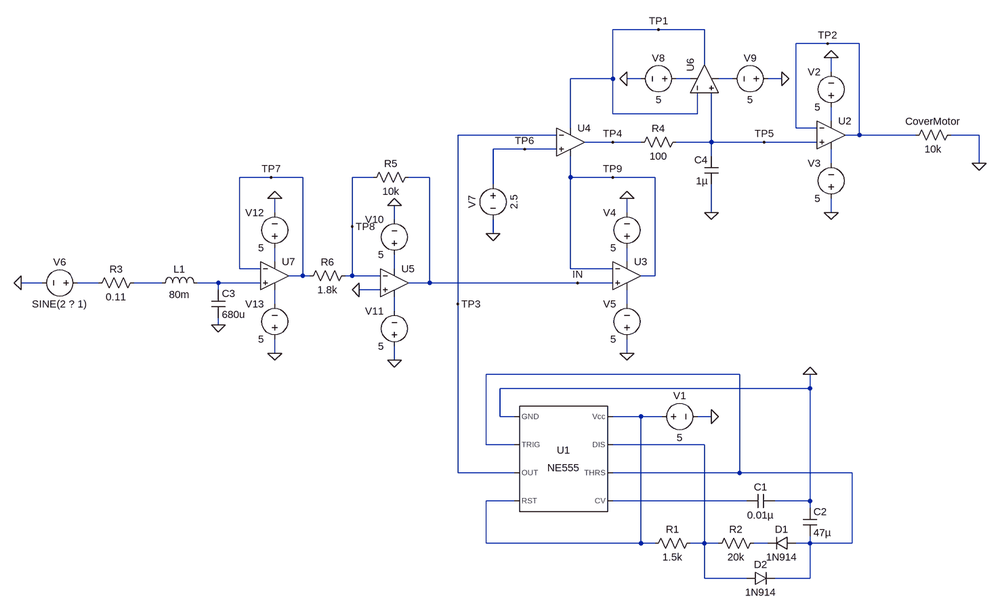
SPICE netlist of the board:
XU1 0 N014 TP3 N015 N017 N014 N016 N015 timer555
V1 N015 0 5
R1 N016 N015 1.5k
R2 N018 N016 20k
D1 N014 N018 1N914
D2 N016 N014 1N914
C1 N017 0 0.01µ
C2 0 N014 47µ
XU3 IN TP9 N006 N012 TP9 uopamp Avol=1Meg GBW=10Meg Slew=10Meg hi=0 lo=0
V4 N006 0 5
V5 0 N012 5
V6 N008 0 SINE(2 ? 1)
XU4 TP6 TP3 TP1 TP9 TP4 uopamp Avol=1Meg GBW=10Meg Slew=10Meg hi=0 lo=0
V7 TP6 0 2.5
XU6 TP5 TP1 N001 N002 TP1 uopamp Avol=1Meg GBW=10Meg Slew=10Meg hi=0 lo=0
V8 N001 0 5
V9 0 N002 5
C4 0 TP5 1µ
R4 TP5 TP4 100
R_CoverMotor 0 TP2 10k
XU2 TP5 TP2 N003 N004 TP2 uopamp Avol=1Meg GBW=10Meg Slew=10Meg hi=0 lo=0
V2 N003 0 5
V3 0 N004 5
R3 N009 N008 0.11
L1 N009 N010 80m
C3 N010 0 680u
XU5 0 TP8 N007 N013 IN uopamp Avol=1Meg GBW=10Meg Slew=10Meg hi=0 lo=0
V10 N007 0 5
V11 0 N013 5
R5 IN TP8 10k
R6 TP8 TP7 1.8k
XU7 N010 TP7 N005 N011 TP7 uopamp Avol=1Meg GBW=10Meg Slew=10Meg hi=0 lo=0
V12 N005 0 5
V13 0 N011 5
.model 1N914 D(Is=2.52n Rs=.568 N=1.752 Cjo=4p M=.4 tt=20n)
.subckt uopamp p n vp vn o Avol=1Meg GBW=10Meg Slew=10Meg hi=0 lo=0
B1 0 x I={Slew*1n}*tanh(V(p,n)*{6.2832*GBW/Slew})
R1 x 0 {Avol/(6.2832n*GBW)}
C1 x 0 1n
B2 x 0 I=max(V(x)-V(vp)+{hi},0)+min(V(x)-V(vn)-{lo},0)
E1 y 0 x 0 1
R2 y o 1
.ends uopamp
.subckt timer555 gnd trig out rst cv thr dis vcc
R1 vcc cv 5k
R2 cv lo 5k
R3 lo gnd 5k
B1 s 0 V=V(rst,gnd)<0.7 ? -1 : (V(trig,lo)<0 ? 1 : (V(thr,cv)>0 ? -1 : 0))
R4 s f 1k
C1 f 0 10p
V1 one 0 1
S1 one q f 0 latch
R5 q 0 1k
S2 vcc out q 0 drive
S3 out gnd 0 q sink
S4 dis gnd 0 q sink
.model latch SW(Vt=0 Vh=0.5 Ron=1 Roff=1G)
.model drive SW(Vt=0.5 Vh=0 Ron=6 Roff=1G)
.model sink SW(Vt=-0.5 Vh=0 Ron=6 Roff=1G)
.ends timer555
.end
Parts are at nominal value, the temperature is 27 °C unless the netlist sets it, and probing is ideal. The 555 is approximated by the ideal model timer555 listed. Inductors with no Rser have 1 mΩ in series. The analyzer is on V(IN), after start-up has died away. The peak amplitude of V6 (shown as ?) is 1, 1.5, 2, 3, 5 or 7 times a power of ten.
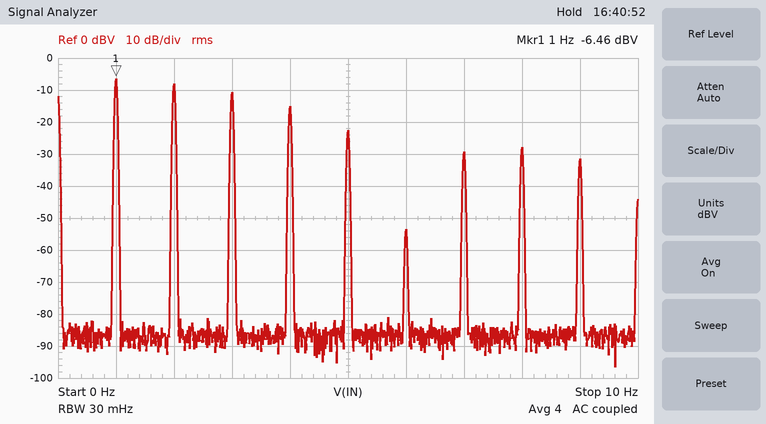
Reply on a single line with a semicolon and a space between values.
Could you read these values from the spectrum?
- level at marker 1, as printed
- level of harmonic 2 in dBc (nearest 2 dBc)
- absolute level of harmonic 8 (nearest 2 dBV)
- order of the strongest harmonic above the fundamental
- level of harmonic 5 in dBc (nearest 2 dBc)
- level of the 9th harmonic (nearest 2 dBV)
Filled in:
-6.46 dBV; -2 dBc; -28 dBV; 2; -16 dBc; -32 dBV
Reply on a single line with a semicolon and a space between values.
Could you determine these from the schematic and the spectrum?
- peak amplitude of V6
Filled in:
1.5 V
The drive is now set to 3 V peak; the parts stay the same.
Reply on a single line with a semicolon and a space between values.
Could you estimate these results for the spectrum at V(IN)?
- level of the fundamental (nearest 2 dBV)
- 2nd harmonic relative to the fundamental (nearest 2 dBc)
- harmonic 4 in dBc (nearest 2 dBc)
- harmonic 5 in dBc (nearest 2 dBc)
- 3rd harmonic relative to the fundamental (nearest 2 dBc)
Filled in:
10 dBV; -4 dBc; -28 dBc; -20 dBc; -14 dBc
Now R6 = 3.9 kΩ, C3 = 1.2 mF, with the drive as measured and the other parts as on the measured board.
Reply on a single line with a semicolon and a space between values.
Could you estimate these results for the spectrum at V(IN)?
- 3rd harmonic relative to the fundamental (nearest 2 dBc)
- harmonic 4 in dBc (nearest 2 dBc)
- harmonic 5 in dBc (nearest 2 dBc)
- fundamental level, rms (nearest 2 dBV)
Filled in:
-38 dBc; -22 dBc; -42 dBc; 2 dBV
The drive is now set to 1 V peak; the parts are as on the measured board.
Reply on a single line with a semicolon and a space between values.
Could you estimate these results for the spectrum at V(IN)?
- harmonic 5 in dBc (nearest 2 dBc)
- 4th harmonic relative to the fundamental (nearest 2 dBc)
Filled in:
-12 dBc; -6 dBc
